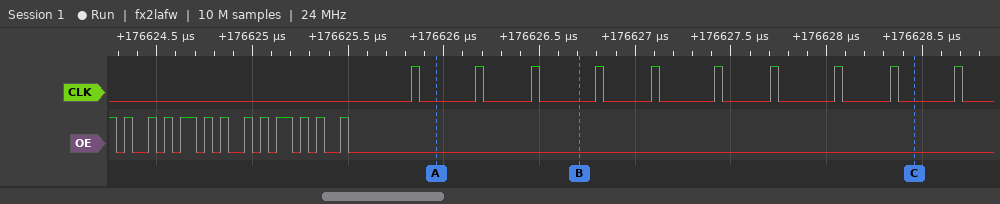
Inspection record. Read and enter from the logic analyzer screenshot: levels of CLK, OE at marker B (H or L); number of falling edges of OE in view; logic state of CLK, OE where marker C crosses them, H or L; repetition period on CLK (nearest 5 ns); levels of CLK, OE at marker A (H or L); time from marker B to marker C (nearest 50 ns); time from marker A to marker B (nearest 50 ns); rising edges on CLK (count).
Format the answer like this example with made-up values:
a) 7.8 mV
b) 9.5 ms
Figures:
a) CLK=L, OE=L
b) 13
c) CLK=L, OE=L
d) 315 ns
e) CLK=L, OE=L
f) 1750 ns
g) 750 ns
h) 10
